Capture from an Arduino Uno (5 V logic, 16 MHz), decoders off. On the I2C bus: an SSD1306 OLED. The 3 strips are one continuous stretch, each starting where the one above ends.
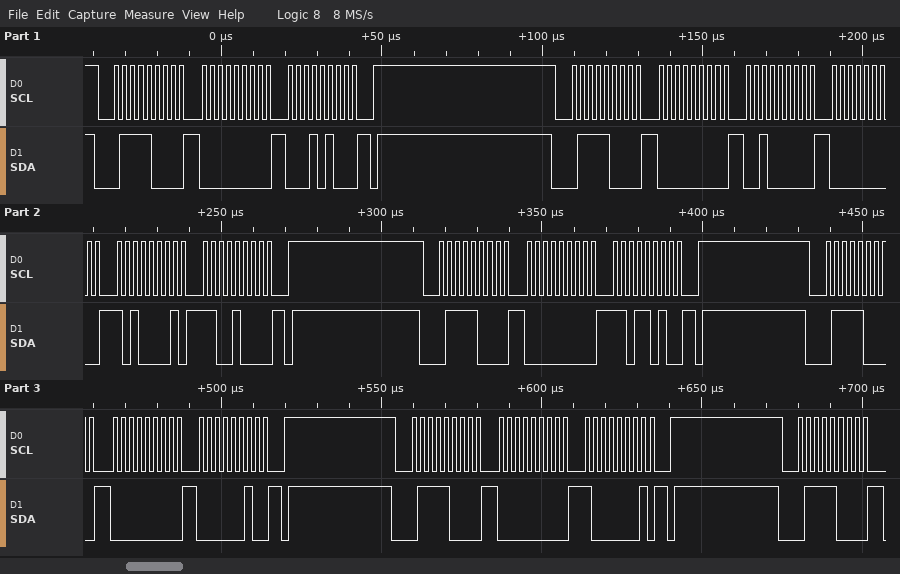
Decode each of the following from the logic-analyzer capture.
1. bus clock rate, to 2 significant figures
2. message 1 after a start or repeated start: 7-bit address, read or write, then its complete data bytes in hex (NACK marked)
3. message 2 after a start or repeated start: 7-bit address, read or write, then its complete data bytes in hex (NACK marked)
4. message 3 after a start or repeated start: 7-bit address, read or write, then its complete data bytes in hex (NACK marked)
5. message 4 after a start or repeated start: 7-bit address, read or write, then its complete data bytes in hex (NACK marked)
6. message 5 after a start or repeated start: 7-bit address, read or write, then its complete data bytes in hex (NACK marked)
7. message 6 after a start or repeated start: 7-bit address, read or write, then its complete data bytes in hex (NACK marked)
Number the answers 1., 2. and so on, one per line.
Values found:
1. 400 kHz
2. 0x3C write: 00 14
3. 0x3C write: 00 20 00 A1 C8
4. 0x3C write: 00 DA
5. 0x3C write: 00 02
6. 0x3C write: 00 81
7. 0x3C write
